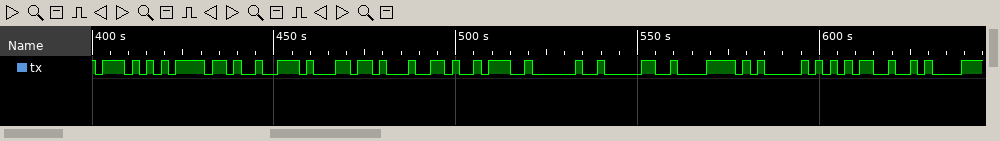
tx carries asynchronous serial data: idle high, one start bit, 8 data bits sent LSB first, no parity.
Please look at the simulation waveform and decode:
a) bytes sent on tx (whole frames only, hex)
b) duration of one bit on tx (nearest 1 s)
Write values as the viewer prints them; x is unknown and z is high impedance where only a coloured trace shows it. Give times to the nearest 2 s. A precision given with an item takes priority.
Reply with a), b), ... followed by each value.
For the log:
a) 57, 6F, 72, 6C, 64, 3A, 20, 30, 78, 41, 35, 0A
b) 2 s
